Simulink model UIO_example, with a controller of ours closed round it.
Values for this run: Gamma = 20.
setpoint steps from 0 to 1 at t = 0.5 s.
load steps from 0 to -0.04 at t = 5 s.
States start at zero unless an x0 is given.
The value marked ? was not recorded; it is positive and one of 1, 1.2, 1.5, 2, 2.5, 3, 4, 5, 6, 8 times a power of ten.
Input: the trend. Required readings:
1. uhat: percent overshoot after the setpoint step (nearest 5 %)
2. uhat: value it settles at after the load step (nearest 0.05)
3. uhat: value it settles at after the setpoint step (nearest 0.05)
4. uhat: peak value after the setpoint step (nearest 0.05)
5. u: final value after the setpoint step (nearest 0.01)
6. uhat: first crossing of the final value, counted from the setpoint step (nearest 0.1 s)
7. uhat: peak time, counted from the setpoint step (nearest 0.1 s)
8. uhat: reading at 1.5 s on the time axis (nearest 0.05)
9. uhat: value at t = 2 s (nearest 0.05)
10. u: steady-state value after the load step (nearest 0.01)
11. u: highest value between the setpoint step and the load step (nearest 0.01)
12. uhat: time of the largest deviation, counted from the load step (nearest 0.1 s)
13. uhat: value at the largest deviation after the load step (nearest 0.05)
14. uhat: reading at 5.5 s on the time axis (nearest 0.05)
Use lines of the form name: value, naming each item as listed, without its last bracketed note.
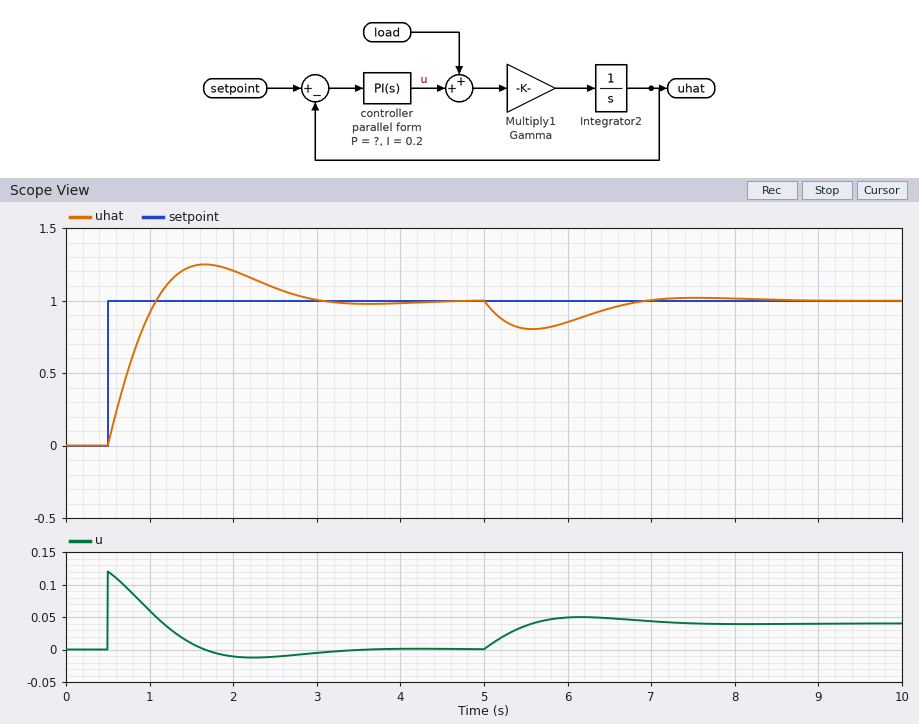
uhat: percent overshoot after the setpoint step: 25 %
uhat: value it settles at after the load step: 1.00
uhat: value it settles at after the setpoint step: 1.00
uhat: peak value after the setpoint step: 1.25
u: final value after the setpoint step: 0.00
uhat: first crossing of the final value, counted from the setpoint step: 0.6 s
uhat: peak time, counted from the setpoint step: 1.2 s
uhat: reading at 1.5 s on the time axis: 1.25
uhat: value at t = 2 s: 1.20
u: steady-state value after the load step: 0.04
u: highest value between the setpoint step and the load step: 0.12
uhat: time of the largest deviation, counted from the load step: 0.6 s
uhat: value at the largest deviation after the load step: 0.80
uhat: reading at 5.5 s on the time axis: 0.80
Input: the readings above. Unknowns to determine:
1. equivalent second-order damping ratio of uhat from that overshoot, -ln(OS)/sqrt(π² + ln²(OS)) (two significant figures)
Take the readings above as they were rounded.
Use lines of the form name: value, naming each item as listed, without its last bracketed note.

equivalent second-order damping ratio of uhat from that overshoot, -ln(OS)/sqrt(π² + ln²(OS)): 0.40
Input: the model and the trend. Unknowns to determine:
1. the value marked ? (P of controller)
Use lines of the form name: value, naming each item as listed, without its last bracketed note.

the value marked ?: 0.12
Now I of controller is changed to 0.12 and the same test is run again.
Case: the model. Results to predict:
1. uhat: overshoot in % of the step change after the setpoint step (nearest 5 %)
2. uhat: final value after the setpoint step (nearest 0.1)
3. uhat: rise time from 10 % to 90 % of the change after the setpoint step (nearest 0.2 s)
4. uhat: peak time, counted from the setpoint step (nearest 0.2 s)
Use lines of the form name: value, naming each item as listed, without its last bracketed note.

uhat: overshoot in % of the step change after the setpoint step: 20 %
uhat: final value after the setpoint step: 1.0
uhat: rise time from 10 % to 90 % of the change after the setpoint step: 0.6 s
uhat: peak time, counted from the setpoint step: 1.4 s
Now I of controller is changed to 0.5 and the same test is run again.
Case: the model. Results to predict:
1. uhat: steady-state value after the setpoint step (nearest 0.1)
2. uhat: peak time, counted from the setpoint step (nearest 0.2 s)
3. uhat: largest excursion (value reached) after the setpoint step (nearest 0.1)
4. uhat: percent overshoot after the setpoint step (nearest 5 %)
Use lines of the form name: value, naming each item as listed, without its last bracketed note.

uhat: steady-state value after the setpoint step: 1.0
uhat: peak time, counted from the setpoint step: 0.8 s
uhat: largest excursion (value reached) after the setpoint step: 1.4
uhat: percent overshoot after the setpoint step: 40 %
